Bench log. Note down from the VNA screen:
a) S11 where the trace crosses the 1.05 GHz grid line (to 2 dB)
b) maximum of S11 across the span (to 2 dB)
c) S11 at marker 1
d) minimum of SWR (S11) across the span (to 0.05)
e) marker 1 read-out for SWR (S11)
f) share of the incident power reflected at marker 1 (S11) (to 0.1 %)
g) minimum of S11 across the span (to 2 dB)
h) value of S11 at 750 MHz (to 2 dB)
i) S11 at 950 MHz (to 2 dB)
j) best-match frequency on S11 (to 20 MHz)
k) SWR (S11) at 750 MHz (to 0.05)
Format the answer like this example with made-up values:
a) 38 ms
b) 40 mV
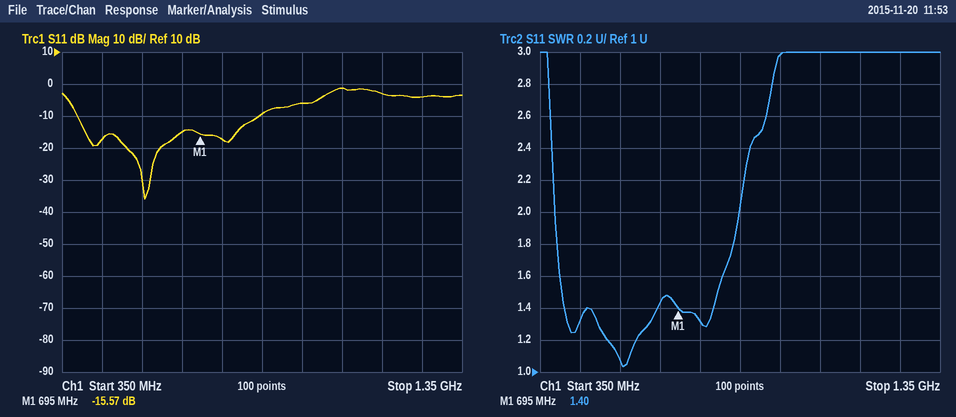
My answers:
a) -2 dB
b) -2 dB
c) -15.57 dB
d) 1.05
e) 1.40
f) 2.8 %
g) -36 dB
h) -18 dB
i) -6 dB
j) 560 MHz
k) 1.30
